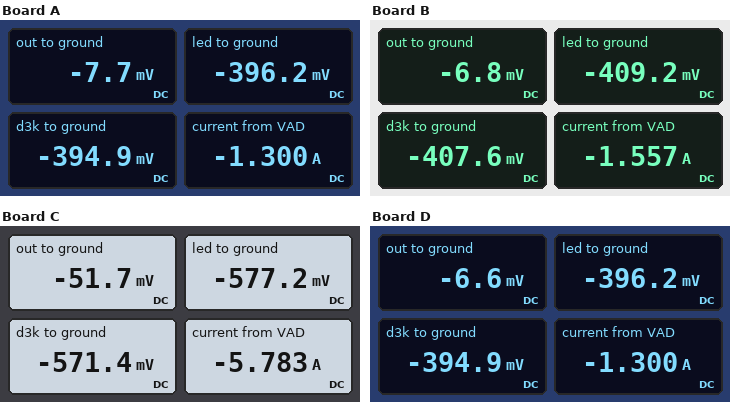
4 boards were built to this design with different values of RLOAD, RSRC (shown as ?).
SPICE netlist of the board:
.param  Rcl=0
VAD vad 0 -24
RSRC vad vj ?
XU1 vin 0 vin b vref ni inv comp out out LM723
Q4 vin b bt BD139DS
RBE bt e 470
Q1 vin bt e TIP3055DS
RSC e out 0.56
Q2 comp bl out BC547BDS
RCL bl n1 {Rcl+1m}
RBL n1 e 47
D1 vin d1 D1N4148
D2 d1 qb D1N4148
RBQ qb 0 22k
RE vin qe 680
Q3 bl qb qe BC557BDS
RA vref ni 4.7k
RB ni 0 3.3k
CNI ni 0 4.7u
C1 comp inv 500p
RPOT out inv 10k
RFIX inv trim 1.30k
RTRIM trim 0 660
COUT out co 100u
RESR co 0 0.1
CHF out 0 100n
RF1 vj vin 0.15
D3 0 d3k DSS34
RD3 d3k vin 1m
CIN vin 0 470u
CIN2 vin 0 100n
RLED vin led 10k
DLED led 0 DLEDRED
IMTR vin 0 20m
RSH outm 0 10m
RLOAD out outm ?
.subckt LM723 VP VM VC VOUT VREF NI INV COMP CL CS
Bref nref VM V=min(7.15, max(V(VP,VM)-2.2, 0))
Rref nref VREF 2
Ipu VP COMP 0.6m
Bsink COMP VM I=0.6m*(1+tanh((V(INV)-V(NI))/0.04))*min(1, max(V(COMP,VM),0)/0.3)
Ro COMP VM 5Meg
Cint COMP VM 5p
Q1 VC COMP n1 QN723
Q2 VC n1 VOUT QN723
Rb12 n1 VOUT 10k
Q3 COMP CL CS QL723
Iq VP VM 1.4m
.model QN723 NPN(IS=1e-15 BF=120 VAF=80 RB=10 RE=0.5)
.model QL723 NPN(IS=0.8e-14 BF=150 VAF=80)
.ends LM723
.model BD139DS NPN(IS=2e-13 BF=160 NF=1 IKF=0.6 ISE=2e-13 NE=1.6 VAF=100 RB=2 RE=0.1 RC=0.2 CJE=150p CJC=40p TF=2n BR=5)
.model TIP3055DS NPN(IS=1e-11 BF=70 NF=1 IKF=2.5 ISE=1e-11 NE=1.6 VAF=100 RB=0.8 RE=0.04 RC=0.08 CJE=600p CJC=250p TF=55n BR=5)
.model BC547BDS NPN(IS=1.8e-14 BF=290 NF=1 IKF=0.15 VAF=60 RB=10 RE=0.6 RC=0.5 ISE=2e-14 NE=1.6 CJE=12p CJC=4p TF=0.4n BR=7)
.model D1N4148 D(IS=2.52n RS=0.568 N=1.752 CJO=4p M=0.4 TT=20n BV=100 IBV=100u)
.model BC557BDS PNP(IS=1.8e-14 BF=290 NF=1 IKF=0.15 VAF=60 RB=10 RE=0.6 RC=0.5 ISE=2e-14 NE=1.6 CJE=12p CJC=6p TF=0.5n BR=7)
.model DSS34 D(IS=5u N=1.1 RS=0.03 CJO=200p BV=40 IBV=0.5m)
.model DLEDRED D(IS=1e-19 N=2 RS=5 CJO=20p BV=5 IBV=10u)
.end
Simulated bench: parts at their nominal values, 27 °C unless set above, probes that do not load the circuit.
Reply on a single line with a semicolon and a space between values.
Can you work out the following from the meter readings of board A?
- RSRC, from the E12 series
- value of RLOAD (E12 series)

18 Ω; 220 Ω
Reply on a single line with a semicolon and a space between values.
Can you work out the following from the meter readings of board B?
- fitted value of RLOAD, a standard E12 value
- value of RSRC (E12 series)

120 Ω; 15 Ω
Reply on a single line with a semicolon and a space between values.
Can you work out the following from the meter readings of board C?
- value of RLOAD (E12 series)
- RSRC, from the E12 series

68 Ω; 3.9 Ω
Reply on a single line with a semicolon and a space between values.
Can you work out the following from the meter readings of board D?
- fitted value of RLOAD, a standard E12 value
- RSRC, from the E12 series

180 Ω; 18 Ω
